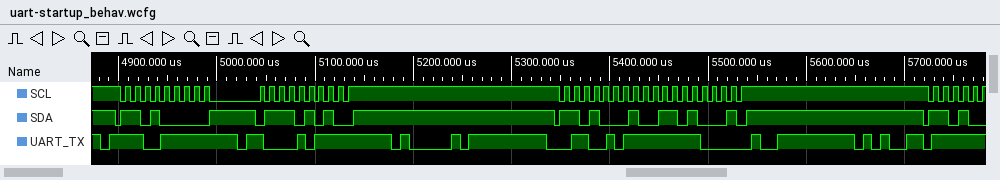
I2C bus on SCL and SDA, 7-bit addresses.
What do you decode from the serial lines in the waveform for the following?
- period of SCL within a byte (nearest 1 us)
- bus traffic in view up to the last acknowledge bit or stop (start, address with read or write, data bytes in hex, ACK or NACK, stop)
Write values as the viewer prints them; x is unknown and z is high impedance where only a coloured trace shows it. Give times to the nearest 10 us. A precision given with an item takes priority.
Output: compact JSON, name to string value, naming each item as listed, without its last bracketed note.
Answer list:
{"period of SCL within a byte": "10 us", "bus traffic in view up to the last acknowledge bit or stop": "start, address 68 write ACK, 75 ACK, stop, start, address 68 read ACK, 68 NACK, stop"}
